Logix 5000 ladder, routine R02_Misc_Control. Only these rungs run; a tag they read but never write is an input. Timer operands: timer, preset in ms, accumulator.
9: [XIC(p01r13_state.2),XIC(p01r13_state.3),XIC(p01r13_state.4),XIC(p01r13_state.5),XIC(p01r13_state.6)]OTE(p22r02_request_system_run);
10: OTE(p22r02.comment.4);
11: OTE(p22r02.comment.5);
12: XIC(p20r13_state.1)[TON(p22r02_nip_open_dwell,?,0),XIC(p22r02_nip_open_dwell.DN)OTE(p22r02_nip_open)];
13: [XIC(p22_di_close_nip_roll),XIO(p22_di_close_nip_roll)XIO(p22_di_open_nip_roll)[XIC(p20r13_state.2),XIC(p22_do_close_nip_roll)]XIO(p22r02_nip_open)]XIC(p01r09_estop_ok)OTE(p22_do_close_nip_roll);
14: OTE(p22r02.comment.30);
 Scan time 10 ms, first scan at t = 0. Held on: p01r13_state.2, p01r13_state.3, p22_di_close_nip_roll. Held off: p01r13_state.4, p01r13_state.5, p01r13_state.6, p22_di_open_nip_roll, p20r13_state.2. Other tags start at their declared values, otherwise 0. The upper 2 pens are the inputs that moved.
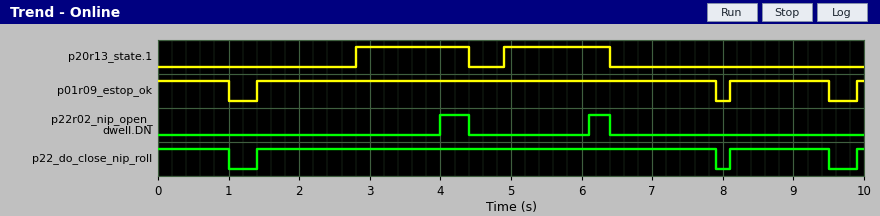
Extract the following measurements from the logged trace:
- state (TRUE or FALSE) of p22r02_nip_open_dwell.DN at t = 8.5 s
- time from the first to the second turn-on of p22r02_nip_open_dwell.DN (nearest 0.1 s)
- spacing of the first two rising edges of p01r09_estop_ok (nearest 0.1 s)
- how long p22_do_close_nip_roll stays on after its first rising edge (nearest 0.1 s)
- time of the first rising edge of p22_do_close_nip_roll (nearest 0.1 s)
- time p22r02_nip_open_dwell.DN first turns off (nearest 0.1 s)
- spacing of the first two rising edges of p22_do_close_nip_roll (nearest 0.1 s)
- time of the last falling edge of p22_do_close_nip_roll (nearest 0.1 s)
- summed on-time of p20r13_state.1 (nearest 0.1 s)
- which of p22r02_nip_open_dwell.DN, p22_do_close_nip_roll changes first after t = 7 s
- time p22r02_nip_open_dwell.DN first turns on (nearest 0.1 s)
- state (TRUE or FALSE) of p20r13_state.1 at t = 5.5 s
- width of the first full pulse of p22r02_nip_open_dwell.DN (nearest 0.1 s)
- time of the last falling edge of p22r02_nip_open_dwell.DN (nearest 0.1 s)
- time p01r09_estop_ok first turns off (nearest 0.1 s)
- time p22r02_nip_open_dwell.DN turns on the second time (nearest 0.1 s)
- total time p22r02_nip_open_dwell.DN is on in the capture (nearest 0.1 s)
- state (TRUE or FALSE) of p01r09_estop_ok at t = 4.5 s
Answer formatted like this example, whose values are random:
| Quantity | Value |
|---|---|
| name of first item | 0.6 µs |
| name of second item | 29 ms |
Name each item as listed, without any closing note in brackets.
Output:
| Quantity | Value |
|---|---|
| state (TRUE or FALSE) of p22r02_nip_open_dwell.DN at t = 8.5 s | FALSE |
| time from the first to the second turn-on of p22r02_nip_open_dwell.DN | 2.1 s |
| spacing of the first two rising edges of p01r09_estop_ok | 6.7 s |
| how long p22_do_close_nip_roll stays on after its first rising edge | 6.5 s |
| time of the first rising edge of p22_do_close_nip_roll | 1.4 s |
| time p22r02_nip_open_dwell.DN first turns off | 4.4 s |
| spacing of the first two rising edges of p22_do_close_nip_roll | 6.7 s |
| time of the last falling edge of p22_do_close_nip_roll | 9.5 s |
| summed on-time of p20r13_state.1 | 3.1 s |
| which of p22r02_nip_open_dwell.DN, p22_do_close_nip_roll changes first after t = 7 s | p22_do_close_nip_roll |
| time p22r02_nip_open_dwell.DN first turns on | 4.0 s |
| state (TRUE or FALSE) of p20r13_state.1 at t = 5.5 s | TRUE |
| width of the first full pulse of p22r02_nip_open_dwell.DN | 0.4 s |
| time of the last falling edge of p22r02_nip_open_dwell.DN | 6.4 s |
| time p01r09_estop_ok first turns off | 1.0 s |
| time p22r02_nip_open_dwell.DN turns on the second time | 6.1 s |
| total time p22r02_nip_open_dwell.DN is on in the capture | 0.7 s |
| state (TRUE or FALSE) of p01r09_estop_ok at t = 4.5 s | TRUE |
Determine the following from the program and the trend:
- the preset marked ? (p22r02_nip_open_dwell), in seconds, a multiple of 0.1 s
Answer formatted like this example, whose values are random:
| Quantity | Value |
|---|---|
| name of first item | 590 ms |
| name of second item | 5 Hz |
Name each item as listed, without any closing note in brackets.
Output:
| Quantity | Value |
|---|---|
| the preset marked ? (p22r02_nip_open_dwell), in seconds, a multiple of 0.1 s | 1.2 s |
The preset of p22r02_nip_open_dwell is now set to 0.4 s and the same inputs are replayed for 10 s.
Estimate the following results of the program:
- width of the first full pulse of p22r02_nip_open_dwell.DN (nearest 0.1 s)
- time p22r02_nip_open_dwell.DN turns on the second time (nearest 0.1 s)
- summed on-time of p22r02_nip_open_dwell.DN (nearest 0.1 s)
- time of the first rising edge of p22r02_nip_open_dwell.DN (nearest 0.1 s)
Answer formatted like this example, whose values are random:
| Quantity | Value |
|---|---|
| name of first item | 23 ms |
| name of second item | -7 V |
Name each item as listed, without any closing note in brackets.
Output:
| Quantity | Value |
|---|---|
| width of the first full pulse of p22r02_nip_open_dwell.DN | 1.2 s |
| time p22r02_nip_open_dwell.DN turns on the second time | 5.3 s |
| summed on-time of p22r02_nip_open_dwell.DN | 2.3 s |
| time of the first rising edge of p22r02_nip_open_dwell.DN | 3.2 s |
